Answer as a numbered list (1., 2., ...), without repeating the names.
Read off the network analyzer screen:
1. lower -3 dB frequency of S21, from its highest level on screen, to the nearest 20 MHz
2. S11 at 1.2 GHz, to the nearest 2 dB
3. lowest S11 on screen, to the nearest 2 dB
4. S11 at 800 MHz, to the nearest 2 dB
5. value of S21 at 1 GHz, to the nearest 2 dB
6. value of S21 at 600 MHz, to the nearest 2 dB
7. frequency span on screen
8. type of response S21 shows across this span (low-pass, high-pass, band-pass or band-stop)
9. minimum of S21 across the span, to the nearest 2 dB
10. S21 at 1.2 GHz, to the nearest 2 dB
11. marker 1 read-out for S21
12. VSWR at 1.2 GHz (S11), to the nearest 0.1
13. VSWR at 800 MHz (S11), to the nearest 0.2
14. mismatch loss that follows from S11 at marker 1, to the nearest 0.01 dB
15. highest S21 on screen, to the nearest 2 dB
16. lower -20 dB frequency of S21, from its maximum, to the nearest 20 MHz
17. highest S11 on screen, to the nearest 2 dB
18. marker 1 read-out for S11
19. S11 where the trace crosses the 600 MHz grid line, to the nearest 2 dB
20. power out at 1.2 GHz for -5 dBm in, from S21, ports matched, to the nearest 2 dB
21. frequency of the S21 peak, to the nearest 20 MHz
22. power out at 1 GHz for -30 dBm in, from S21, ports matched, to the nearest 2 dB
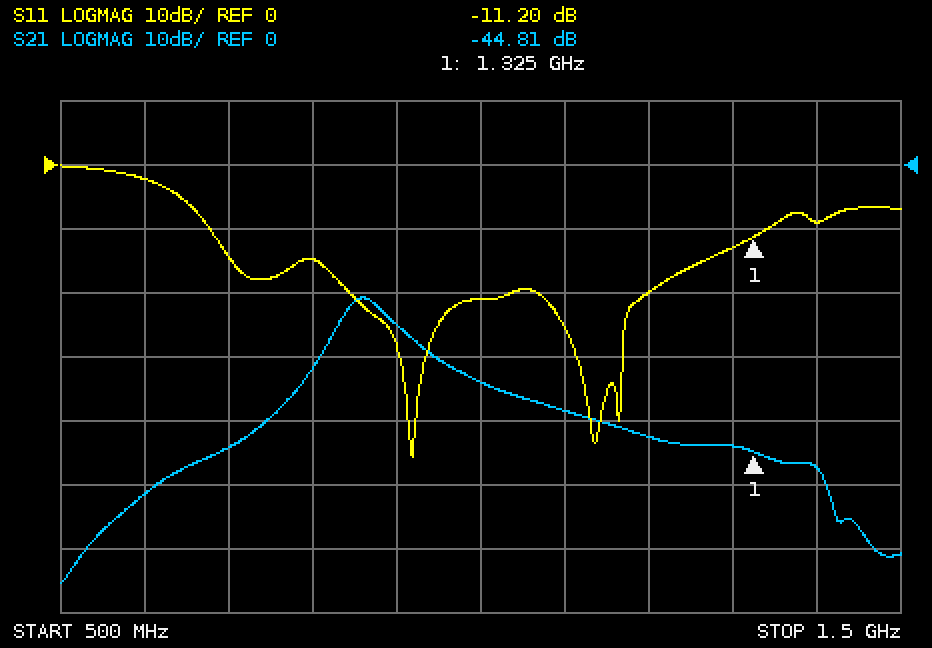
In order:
1. 840 MHz
2. -20 dB
3. -46 dB
4. -14 dB
5. -34 dB
6. -52 dB
7. 1 GHz
8. band-pass
9. -66 dB
10. -42 dB
11. -44.81 dB
12. 1.2
13. 1.4
14. 0.34 dB
15. -20 dB
16. 740 MHz
17. 0 dB
18. -11.20 dB
19. -2 dB
20. -48 dBm
21. 860 MHz
22. -64 dBm
